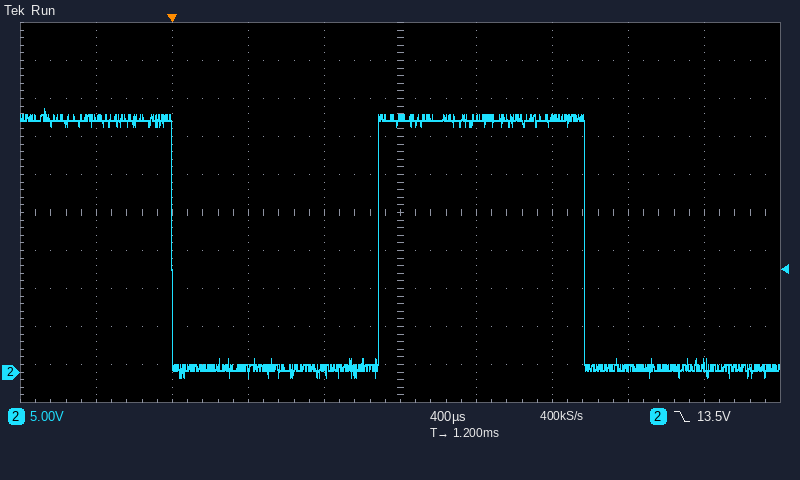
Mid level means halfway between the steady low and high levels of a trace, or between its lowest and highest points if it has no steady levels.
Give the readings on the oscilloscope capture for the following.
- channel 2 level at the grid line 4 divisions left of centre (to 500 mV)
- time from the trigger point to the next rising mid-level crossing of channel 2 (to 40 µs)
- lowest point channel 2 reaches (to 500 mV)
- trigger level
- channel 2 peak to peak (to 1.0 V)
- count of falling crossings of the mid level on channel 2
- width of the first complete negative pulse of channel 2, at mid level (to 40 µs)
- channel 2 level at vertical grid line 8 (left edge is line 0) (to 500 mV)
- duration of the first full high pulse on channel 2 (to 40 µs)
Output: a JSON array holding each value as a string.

["33.5 V", "1.08 ms", "-500 mV", "13.5 V", "35.0 V", "2", "1.08 ms", "500 mV", "1.08 ms"]
